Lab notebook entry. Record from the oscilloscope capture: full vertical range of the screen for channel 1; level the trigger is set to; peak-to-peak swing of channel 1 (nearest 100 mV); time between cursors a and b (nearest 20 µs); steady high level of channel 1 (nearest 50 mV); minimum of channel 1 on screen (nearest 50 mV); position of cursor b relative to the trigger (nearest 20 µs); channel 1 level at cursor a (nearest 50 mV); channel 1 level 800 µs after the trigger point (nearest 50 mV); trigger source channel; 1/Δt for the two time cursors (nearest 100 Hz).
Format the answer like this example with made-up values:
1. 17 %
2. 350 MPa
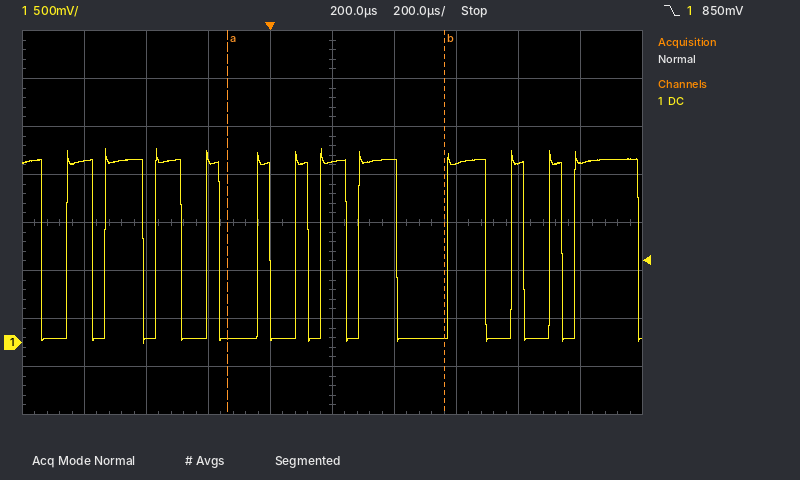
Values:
1. 4 V
2. 850 mV
3. 2.00 V
4. 700 µs
5. 1.90 V
6. 0 mV
7. +560 µs
8. 50 mV
9. 1.85 V
10. channel 1
11. 1.4 kHz
